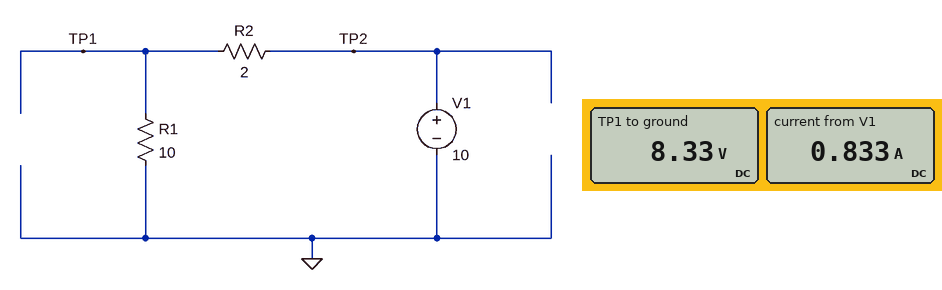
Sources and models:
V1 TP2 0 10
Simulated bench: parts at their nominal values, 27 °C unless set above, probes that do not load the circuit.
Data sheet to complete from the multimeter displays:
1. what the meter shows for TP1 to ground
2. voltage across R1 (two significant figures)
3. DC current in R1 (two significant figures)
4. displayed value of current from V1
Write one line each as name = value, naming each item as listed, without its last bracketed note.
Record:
what the meter shows for TP1 to ground = 8.33 V
voltage across R1 = 8.3 V
DC current in R1 = 830 mA
displayed value of current from V1 = 0.833 A
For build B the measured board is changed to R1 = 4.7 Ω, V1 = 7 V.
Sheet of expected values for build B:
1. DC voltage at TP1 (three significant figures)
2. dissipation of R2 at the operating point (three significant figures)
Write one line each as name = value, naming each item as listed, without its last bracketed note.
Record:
DC voltage at TP1 = 4.91 V
dissipation of R2 at the operating point = 2.18 W
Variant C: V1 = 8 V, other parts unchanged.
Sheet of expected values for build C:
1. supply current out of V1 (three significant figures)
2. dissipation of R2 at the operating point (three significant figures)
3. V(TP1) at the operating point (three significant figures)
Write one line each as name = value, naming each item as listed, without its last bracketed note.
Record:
supply current out of V1 = 667 mA
dissipation of R2 at the operating point = 889 mW
V(TP1) at the operating point = 6.67 V
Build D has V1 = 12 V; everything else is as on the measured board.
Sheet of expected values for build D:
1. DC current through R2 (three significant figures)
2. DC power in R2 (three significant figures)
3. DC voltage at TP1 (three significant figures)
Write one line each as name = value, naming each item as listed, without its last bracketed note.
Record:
DC current through R2 = 1.00 A
DC power in R2 = 2.00 W
DC voltage at TP1 = 10.0 V
